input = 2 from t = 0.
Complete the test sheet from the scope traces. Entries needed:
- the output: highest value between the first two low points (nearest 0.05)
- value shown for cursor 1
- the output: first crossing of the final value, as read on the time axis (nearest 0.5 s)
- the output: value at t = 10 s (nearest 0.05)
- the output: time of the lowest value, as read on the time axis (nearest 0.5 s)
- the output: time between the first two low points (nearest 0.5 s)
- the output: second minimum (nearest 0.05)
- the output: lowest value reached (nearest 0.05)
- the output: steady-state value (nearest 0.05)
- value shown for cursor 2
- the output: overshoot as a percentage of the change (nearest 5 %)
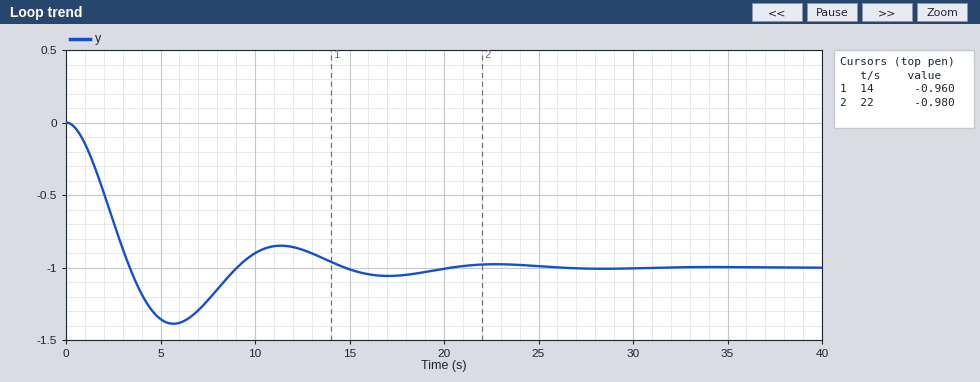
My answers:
-0.85
-0.960
3.5 s
-0.90
5.5 s
11.5 s
-1.05
-1.40
-1.00
-0.980
40 %
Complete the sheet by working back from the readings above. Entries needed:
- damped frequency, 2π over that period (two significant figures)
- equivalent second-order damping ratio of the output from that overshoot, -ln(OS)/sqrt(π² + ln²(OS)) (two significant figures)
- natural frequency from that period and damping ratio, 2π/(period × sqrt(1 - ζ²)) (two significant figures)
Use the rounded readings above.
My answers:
0.55 rad/s
0.28
0.57 rad/s
